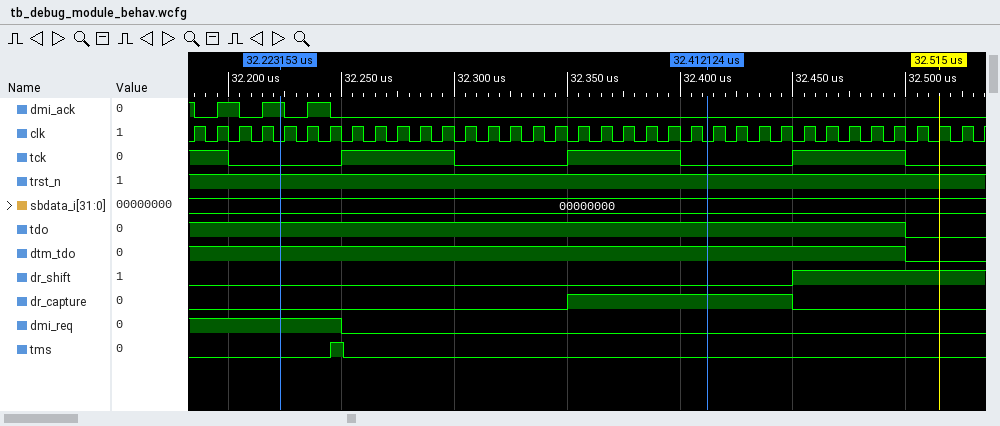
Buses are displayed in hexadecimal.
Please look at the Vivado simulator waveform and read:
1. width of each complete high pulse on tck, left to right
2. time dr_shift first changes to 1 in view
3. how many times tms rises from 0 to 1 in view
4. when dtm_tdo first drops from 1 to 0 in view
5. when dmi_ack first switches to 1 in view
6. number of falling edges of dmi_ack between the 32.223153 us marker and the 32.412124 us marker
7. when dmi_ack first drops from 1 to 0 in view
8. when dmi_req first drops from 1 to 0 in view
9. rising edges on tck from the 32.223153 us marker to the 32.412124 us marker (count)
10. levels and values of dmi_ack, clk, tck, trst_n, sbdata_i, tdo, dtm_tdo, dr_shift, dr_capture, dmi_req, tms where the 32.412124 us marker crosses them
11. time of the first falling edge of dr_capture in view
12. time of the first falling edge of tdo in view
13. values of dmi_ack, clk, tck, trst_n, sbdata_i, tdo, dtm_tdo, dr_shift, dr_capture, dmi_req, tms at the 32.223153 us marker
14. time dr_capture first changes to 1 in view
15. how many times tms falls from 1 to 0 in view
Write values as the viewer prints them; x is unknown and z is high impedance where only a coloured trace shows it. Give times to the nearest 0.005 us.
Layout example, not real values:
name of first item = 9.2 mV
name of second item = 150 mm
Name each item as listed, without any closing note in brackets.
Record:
width of each complete high pulse on tck, left to right = 0.05 us, 0.05 us, 0.05 us
time dr_shift first changes to 1 in view = 32.45 us
how many times tms rises from 0 to 1 in view = 1
when dtm_tdo first drops from 1 to 0 in view = 32.5 us
when dmi_ack first switches to 1 in view = 32.195 us
number of falling edges of dmi_ack between the 32.223153 us marker and the 32.412124 us marker = 2
when dmi_ack first drops from 1 to 0 in view = 32.185 us
when dmi_req first drops from 1 to 0 in view = 32.25 us
rising edges on tck from the 32.223153 us marker to the 32.412124 us marker = 2
levels and values of dmi_ack, clk, tck, trst_n, sbdata_i, tdo, dtm_tdo, dr_shift, dr_capture, dmi_req, tms where the 32.412124 us marker crosses them = dmi_ack=0, clk=0, tck=0, trst_n=1, sbdata_i=00000000, tdo=1, dtm_tdo=1, dr_shift=0, dr_capture=1, dmi_req=0, tms=0
time of the first falling edge of dr_capture in view = 32.45 us
time of the first falling edge of tdo in view = 32.5 us
values of dmi_ack, clk, tck, trst_n, sbdata_i, tdo, dtm_tdo, dr_shift, dr_capture, dmi_req, tms at the 32.223153 us marker = dmi_ack=1, clk=0, tck=0, trst_n=1, sbdata_i=00000000, tdo=1, dtm_tdo=1, dr_shift=0, dr_capture=0, dmi_req=1, tms=0
time dr_capture first changes to 1 in view = 32.35 us
how many times tms falls from 1 to 0 in view = 1
